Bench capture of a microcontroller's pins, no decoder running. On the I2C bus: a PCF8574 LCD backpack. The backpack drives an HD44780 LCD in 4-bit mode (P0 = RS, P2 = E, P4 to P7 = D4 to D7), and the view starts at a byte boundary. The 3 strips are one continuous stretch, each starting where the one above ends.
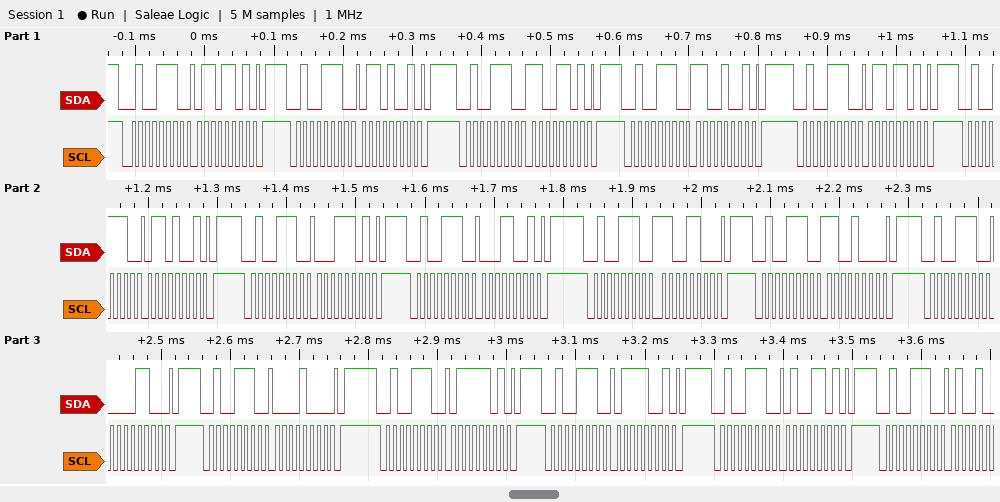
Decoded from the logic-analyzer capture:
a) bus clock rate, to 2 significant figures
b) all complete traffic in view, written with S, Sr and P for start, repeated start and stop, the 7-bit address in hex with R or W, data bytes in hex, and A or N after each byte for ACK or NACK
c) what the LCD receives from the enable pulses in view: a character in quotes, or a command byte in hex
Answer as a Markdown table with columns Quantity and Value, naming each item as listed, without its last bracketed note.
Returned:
| Quantity | Value |
|---|---|
| bus clock rate, to 2 significant figures | 100 kHz |
| all complete traffic in view, written with S, Sr and P for start, repeated start and stop, the 7-bit address in hex with R or W, data bytes in hex, and A or N after each byte for ACK or NACK | S 27W A 6D A P S 27W A 69 A P S 27W A CD A P S 27W A C9 A P S 27W A 6D A P S 27W A 69 A P S 27W A 1D A P S 27W A 19 A P S 27W A CC A P S 27W A C8 A P S 27W A 0C A P S 27W A 08 A P S 27W A 7D A P S 27W A 79 A P S 27W A 4D A P S 27W A |
| what the LCD receives from the enable pulses in view: a character in quotes, or a command byte in hex | 'l' 'a' 0xC0 |
